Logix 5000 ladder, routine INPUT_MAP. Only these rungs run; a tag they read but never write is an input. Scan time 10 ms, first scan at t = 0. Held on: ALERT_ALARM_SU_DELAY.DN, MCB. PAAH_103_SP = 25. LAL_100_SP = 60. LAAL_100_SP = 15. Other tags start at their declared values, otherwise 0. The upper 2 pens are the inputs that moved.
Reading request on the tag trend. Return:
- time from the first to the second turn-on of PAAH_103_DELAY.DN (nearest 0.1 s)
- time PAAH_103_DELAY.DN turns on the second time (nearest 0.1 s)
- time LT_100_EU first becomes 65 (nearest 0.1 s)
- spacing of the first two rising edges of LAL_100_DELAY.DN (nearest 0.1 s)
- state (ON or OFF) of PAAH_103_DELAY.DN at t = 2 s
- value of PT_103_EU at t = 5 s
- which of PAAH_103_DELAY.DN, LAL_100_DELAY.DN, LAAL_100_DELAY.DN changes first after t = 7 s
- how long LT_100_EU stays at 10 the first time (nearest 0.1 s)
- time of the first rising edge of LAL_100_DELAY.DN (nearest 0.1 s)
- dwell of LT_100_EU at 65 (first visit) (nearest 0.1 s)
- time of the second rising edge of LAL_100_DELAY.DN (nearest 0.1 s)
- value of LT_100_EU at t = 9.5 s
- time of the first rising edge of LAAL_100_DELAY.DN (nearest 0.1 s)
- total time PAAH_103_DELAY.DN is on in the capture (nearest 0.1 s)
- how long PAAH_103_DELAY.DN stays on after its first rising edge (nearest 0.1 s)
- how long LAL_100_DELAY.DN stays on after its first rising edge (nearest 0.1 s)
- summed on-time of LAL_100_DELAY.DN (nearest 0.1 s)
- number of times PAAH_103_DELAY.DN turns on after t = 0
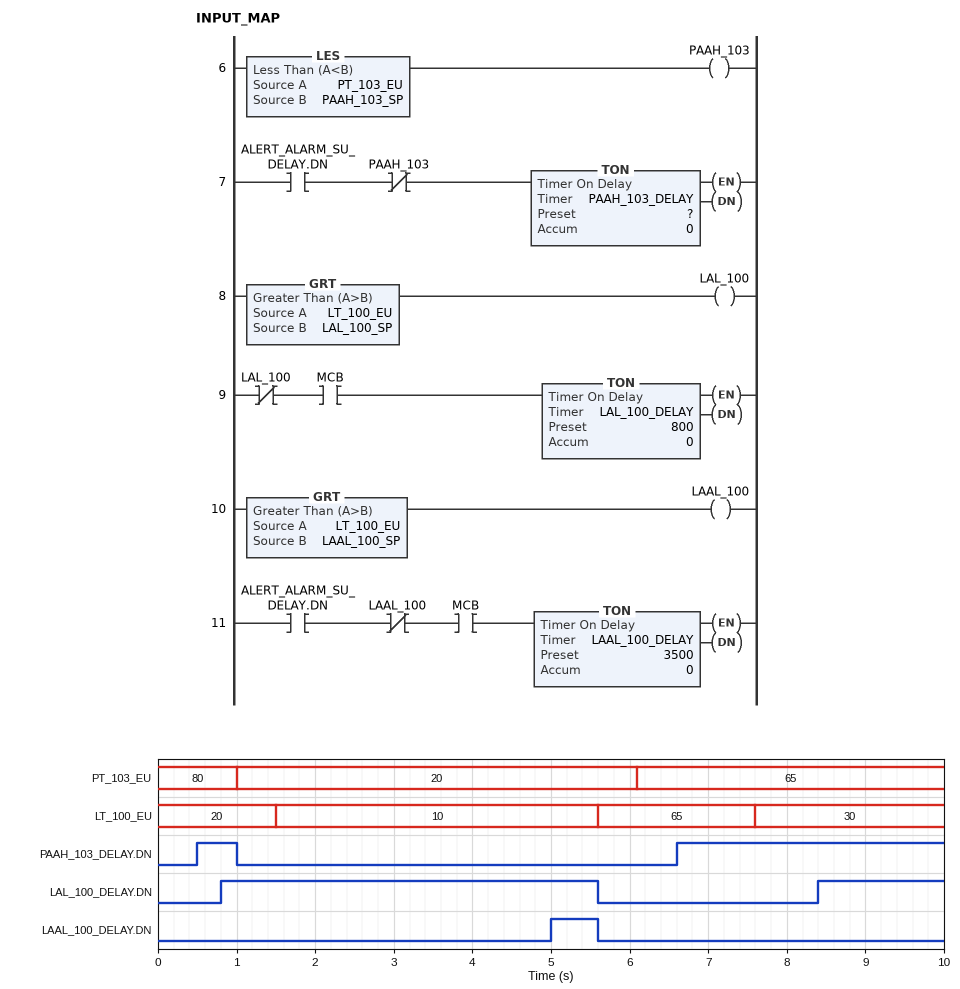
6.1 s
6.6 s
5.6 s
7.6 s
OFF
20
LAL_100_DELAY.DN
4.1 s
0.8 s
2.0 s
8.4 s
30
5.0 s
3.9 s
0.5 s
4.8 s
6.4 s
2
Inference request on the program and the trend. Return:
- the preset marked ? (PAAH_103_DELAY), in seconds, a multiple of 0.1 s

0.5 s
